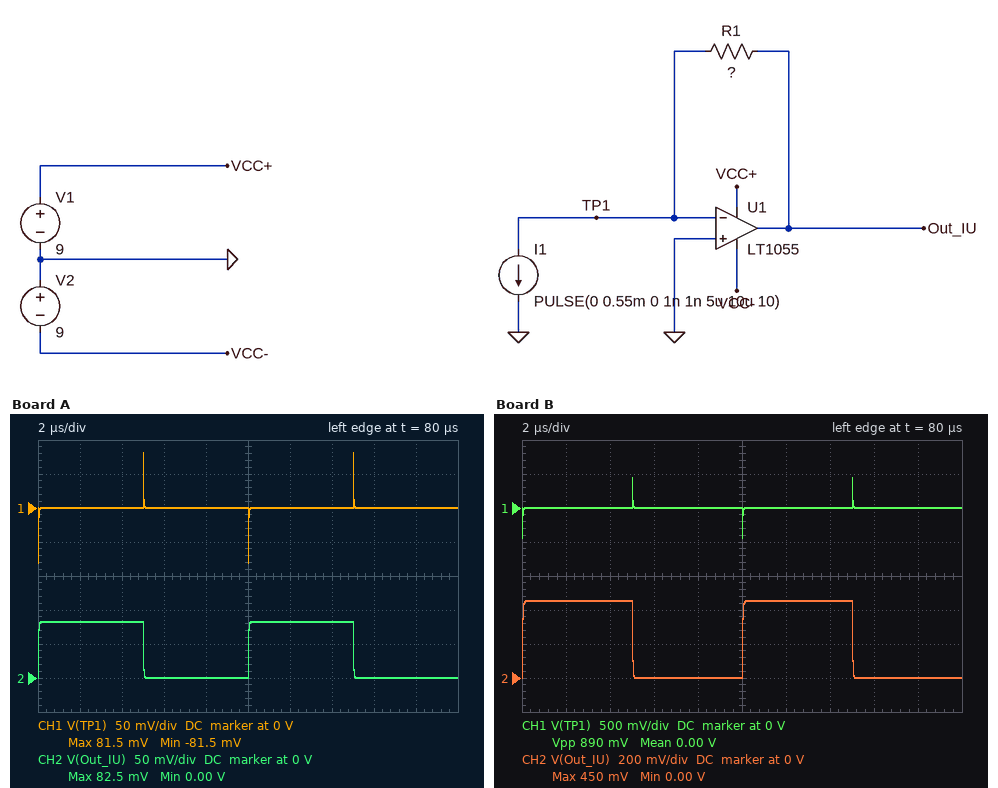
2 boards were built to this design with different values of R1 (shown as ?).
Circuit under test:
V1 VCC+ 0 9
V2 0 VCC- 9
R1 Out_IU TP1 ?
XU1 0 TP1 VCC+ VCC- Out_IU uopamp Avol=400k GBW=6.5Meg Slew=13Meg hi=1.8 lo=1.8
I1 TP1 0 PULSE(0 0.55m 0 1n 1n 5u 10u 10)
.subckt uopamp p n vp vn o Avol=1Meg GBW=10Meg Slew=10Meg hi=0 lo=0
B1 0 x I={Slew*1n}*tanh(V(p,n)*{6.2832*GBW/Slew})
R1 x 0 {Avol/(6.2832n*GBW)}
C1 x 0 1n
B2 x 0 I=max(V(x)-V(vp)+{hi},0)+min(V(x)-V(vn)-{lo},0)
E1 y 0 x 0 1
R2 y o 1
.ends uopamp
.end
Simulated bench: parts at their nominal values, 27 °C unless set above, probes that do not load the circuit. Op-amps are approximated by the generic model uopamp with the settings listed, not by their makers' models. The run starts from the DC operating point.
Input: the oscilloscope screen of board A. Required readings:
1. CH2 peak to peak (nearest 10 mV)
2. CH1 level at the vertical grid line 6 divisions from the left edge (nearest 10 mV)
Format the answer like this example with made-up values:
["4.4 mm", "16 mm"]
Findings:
["80 mV", "0 V"]
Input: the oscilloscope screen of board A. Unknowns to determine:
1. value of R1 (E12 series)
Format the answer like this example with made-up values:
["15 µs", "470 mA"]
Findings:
["150 Ω"]
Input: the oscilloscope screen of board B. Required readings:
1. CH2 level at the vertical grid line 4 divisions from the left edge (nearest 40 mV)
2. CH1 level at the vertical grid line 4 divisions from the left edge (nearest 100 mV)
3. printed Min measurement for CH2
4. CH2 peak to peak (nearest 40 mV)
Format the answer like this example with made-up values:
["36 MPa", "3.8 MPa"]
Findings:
["0 V", "0 V", "0.00 V", "440 mV"]
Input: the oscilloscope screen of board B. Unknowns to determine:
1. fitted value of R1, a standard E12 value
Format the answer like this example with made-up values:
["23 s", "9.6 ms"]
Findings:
["820 Ω"]
